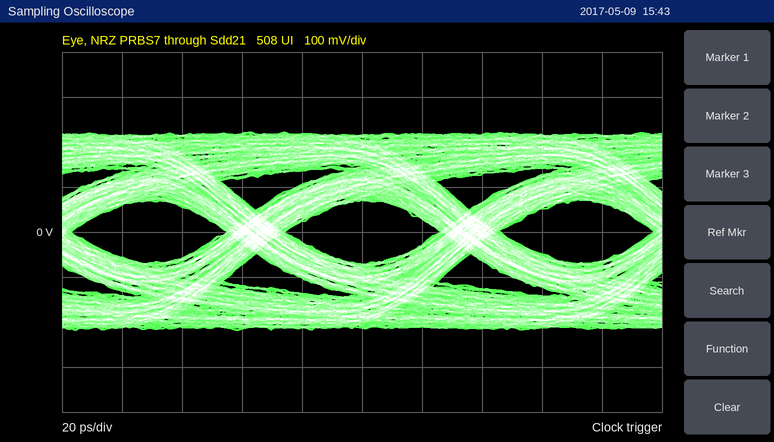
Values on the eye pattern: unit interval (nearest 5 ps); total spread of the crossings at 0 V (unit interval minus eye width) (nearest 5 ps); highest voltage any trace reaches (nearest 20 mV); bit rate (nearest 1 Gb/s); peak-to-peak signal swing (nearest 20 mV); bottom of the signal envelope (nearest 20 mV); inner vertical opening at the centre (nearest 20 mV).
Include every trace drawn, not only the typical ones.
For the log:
70 ps
20 ps
220 mV
14 Gb/s
440 mV
-220 mV
140 mV
